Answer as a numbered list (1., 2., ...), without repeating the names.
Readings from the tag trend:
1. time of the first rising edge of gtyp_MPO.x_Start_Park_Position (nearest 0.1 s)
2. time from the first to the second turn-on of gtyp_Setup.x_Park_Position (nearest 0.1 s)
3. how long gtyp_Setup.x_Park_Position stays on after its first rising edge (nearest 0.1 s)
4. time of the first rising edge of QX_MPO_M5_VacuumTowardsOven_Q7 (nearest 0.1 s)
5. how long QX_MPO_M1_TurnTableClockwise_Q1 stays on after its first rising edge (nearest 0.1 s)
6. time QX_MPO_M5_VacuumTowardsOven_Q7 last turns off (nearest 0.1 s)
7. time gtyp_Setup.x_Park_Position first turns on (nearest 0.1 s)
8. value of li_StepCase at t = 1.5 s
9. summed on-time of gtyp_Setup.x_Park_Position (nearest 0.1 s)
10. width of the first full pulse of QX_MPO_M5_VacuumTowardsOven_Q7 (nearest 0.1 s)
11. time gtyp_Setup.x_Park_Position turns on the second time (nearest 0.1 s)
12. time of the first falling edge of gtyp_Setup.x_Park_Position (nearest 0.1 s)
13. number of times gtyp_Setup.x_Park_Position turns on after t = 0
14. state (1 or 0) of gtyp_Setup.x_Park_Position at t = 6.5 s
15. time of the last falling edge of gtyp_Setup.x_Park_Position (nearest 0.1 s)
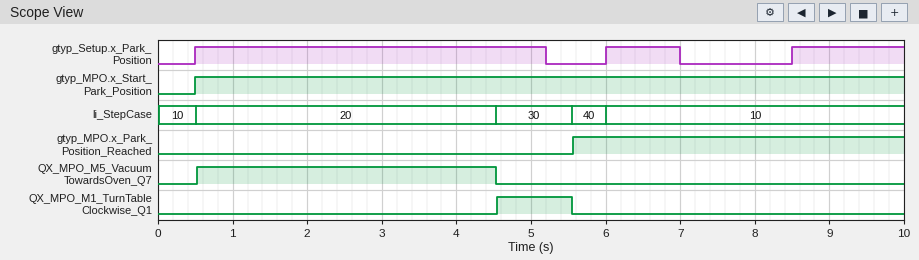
1. 0.5 s
2. 5.5 s
3. 4.7 s
4. 0.5 s
5. 1.0 s
6. 4.5 s
7. 0.5 s
8. 20
9. 7.2 s
10. 4.0 s
11. 6.0 s
12. 5.2 s
13. 3
14. 1
15. 7.0 s
